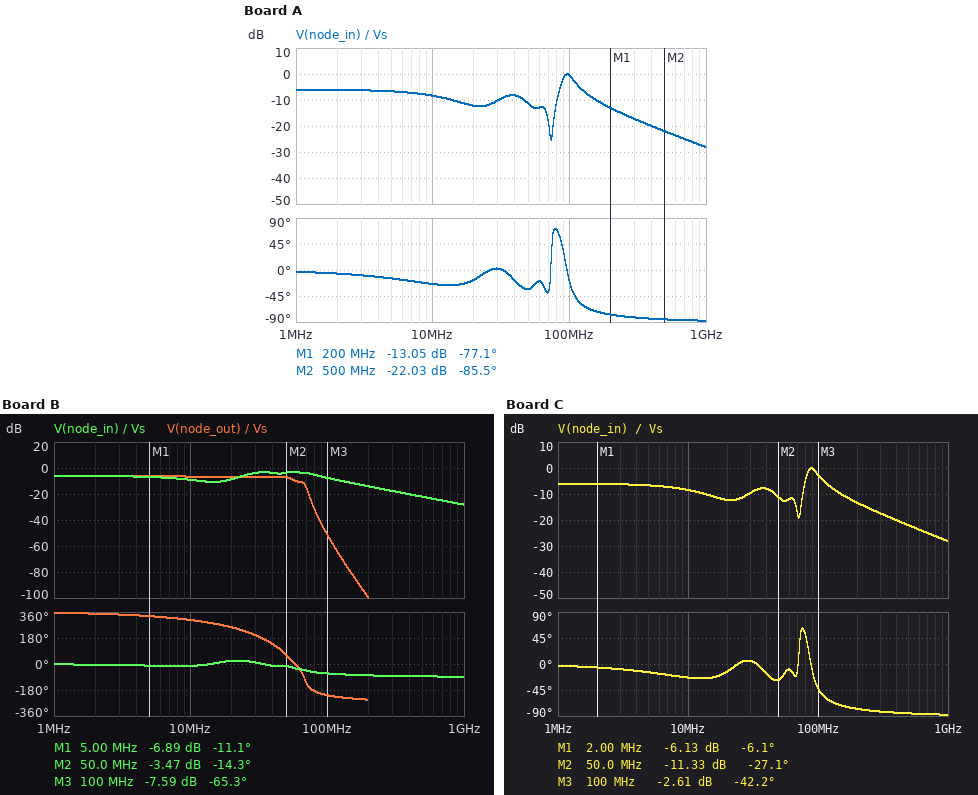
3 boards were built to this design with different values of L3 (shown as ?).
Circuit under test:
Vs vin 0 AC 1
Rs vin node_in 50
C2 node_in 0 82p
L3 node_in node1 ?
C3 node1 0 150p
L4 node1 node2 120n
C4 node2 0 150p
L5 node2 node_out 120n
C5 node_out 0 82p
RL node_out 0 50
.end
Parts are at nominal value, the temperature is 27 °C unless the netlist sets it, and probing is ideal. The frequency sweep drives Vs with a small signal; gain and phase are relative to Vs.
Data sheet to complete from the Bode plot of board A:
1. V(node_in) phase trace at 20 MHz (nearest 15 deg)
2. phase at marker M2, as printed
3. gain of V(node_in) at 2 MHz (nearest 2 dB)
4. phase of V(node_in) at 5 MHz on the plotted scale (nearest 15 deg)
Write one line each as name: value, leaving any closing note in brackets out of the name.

V(node_in) phase trace at 20 MHz: -15 deg
phase at marker M2, as printed: -85.5 deg
gain of V(node_in) at 2 MHz: -6 dB
phase of V(node_in) at 5 MHz on the plotted scale: -15 deg
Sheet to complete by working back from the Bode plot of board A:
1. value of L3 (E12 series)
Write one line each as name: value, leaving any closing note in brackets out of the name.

value of L3: 56 nH
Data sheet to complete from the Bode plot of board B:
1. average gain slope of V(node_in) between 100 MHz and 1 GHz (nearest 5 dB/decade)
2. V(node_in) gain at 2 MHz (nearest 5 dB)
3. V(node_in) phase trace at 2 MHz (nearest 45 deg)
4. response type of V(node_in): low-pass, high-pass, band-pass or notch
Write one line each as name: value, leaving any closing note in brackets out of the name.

average gain slope of V(node_in) between 100 MHz and 1 GHz: -20 dB/decade
V(node_in) gain at 2 MHz: -5 dB
V(node_in) phase trace at 2 MHz: 0 deg
response type of V(node_in): low-pass, high-pass, band-pass or notch: low-pass
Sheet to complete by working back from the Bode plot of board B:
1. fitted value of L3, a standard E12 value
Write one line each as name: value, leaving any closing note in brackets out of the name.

fitted value of L3, a standard E12 value: 220 nH
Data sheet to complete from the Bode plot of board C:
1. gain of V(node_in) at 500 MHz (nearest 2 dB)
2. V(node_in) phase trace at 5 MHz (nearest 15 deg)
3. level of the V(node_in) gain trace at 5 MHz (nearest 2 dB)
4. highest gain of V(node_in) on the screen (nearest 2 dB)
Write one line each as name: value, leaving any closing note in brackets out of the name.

gain of V(node_in) at 500 MHz: -22 dB
V(node_in) phase trace at 5 MHz: -15 deg
level of the V(node_in) gain trace at 5 MHz: -6 dB
highest gain of V(node_in) on the screen: 0 dB
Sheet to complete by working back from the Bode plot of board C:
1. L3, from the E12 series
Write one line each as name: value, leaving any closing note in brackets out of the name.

L3, from the E12 series: 68 nH
